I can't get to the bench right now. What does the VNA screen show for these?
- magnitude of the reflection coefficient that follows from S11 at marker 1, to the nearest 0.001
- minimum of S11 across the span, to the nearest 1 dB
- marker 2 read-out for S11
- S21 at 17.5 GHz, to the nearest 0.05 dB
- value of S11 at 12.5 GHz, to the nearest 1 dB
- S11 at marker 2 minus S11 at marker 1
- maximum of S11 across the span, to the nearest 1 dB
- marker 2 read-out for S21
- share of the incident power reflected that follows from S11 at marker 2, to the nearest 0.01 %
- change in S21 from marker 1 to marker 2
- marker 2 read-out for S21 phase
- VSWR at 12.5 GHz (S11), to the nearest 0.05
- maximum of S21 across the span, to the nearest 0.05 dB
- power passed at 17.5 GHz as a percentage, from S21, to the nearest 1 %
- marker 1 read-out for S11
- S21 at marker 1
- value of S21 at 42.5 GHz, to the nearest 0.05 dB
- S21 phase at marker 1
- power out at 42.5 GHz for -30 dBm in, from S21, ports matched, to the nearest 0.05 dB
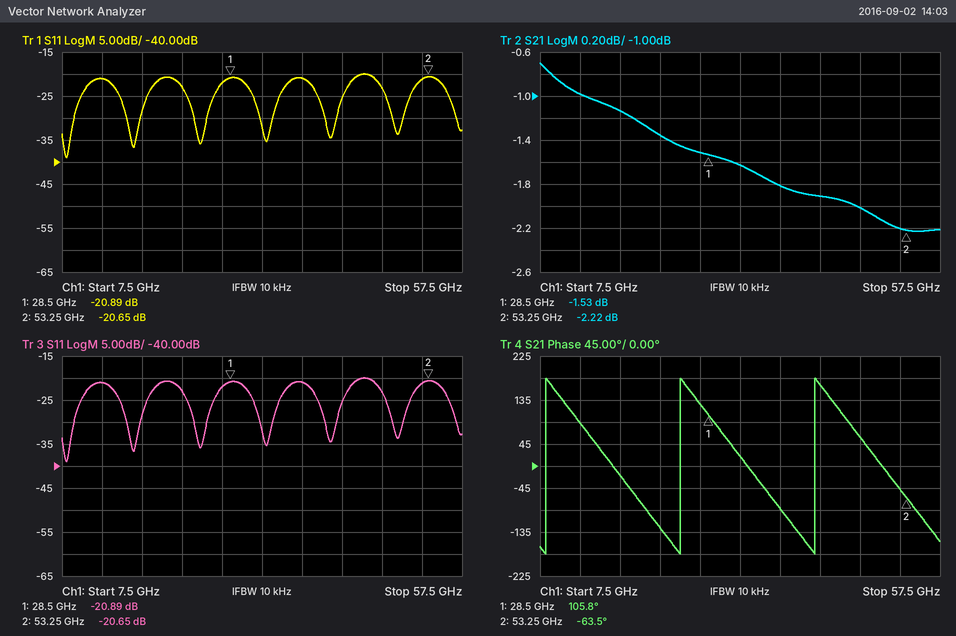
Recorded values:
0.090
-39 dB
-20.65 dB
-1.15 dB
-21 dB
0.24 dB
-20 dB
-2.22 dB
0.86 %
-0.69 dB
-63.5°
1.20
-0.70 dB
77 %
-20.89 dB
-1.53 dB
-1.90 dB
105.8°
-31.90 dBm
